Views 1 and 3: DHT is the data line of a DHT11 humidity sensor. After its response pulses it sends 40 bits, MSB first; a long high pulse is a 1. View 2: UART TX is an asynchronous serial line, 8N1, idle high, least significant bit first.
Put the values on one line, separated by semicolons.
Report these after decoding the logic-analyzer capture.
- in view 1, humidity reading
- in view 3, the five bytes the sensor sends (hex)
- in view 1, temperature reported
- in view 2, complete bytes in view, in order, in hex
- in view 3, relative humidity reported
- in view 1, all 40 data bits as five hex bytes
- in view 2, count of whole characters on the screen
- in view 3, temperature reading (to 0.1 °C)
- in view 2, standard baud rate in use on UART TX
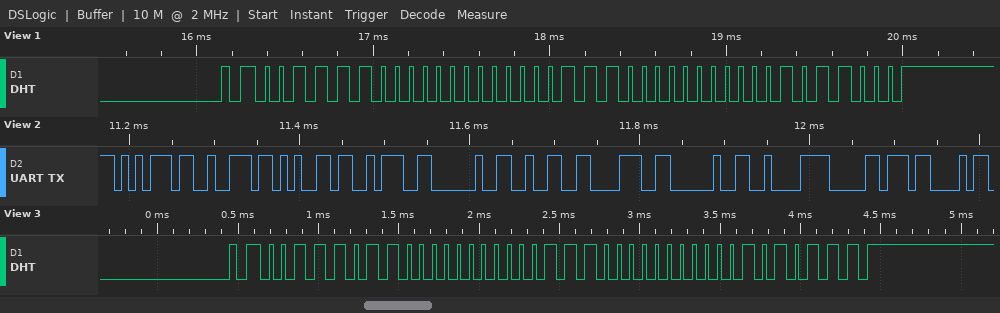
60 %; 3B 00 1C 00 57; 28.0 °C; 75 72 65 3A 20 32 38 20 C2 B0 43; 59 %; 3C 00 1C 00 58; 11; 28.0 °C; 115200 baud
